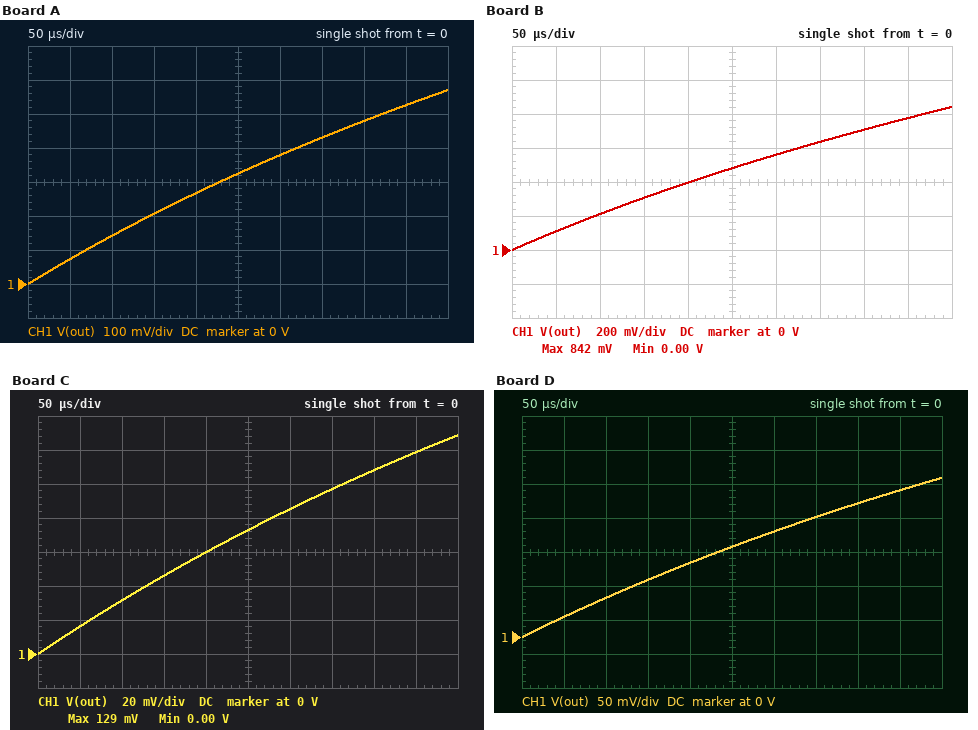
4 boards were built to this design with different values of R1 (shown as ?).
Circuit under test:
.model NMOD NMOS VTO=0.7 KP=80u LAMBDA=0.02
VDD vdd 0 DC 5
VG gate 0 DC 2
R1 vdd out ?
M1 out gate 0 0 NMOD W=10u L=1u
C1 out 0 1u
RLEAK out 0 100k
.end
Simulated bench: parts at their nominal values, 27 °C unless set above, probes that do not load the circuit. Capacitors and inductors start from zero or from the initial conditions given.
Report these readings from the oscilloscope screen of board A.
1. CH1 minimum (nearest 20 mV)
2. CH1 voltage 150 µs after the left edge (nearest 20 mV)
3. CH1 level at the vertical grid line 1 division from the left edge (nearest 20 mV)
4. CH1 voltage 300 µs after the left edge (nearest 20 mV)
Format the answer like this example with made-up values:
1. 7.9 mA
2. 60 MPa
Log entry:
1. 0 V
2. 200 mV
3. 80 mV
4. 380 mV
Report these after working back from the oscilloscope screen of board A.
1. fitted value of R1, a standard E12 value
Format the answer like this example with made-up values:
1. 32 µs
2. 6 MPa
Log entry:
1. 3.3 kΩ
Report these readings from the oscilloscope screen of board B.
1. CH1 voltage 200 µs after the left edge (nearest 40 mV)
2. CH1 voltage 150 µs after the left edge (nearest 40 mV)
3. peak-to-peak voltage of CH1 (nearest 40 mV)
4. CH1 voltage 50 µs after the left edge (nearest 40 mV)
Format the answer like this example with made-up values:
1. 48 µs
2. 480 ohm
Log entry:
1. 400 mV
2. 320 mV
3. 840 mV
4. 120 mV
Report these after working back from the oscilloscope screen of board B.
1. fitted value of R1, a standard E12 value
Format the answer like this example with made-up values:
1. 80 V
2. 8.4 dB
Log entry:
1. 2.2 kΩ
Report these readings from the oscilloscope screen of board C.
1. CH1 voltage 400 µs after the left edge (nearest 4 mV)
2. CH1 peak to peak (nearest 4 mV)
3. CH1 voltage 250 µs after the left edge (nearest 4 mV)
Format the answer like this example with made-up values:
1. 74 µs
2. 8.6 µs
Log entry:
1. 108 mV
2. 128 mV
3. 72 mV
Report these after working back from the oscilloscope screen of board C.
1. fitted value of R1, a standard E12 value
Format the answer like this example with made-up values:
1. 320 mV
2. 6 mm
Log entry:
1. 15 kΩ
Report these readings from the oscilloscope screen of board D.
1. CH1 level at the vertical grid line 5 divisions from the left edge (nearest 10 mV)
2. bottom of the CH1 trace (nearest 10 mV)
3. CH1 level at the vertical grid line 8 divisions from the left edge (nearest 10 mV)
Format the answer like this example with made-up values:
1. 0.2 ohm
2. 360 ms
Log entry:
1. 130 mV
2. 0 V
3. 200 mV
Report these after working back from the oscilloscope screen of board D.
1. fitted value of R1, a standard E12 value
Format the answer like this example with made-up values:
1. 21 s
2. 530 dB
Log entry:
1. 8.2 kΩ
